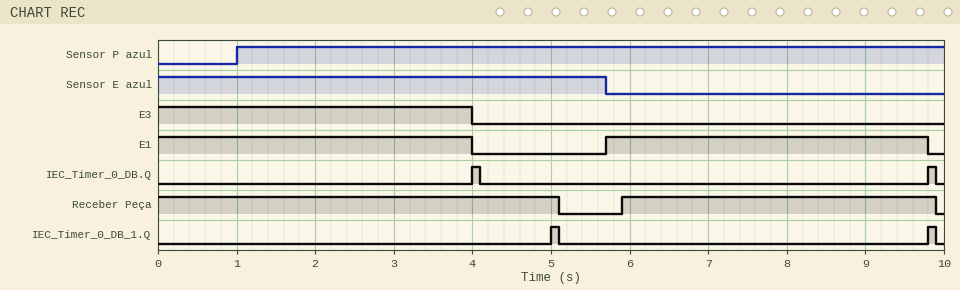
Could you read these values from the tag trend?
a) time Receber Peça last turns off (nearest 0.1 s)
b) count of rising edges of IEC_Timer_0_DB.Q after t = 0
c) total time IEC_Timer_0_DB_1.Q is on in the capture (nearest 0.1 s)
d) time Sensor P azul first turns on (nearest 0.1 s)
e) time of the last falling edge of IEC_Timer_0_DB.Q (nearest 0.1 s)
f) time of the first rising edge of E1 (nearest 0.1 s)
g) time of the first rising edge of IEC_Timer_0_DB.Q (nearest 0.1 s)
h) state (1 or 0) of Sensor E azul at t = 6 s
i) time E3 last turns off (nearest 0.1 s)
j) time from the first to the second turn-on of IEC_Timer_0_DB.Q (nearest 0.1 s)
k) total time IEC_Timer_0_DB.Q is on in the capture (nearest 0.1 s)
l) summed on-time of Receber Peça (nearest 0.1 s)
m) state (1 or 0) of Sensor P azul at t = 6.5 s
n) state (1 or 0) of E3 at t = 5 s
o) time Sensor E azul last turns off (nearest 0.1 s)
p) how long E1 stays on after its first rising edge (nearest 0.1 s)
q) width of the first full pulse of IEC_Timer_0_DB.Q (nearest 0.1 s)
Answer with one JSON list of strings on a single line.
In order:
["9.9 s", "2", "0.2 s", "1.0 s", "9.9 s", "5.7 s", "4.0 s", "0", "4.0 s", "5.8 s", "0.2 s", "9.1 s", "1", "0", "5.7 s", "4.1 s", "0.1 s"]
